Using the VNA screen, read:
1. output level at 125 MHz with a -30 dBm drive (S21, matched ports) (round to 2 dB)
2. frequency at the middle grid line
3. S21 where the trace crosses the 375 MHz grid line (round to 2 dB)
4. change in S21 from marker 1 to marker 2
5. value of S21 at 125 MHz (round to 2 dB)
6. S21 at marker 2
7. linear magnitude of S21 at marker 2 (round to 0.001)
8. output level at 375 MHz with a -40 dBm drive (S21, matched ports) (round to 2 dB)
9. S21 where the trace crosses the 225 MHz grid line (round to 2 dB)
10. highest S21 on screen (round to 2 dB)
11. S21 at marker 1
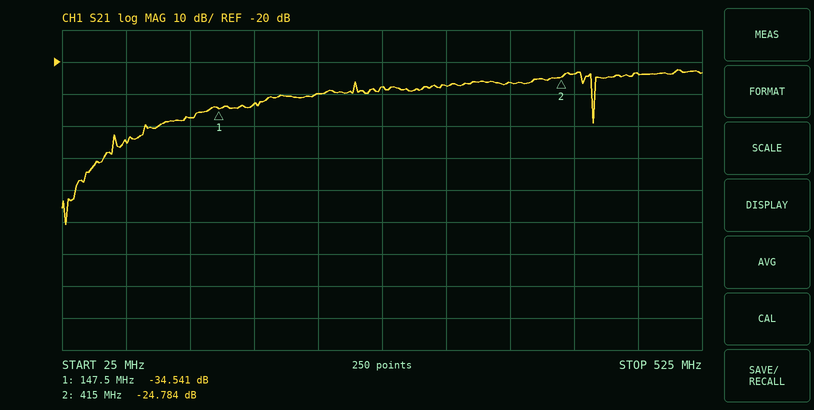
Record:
-68 dBm
275 MHz
-26 dB
9.757 dB
-38 dB
-24.784 dB
0.058
-66 dBm
-30 dB
-22 dB
-34.541 dB
